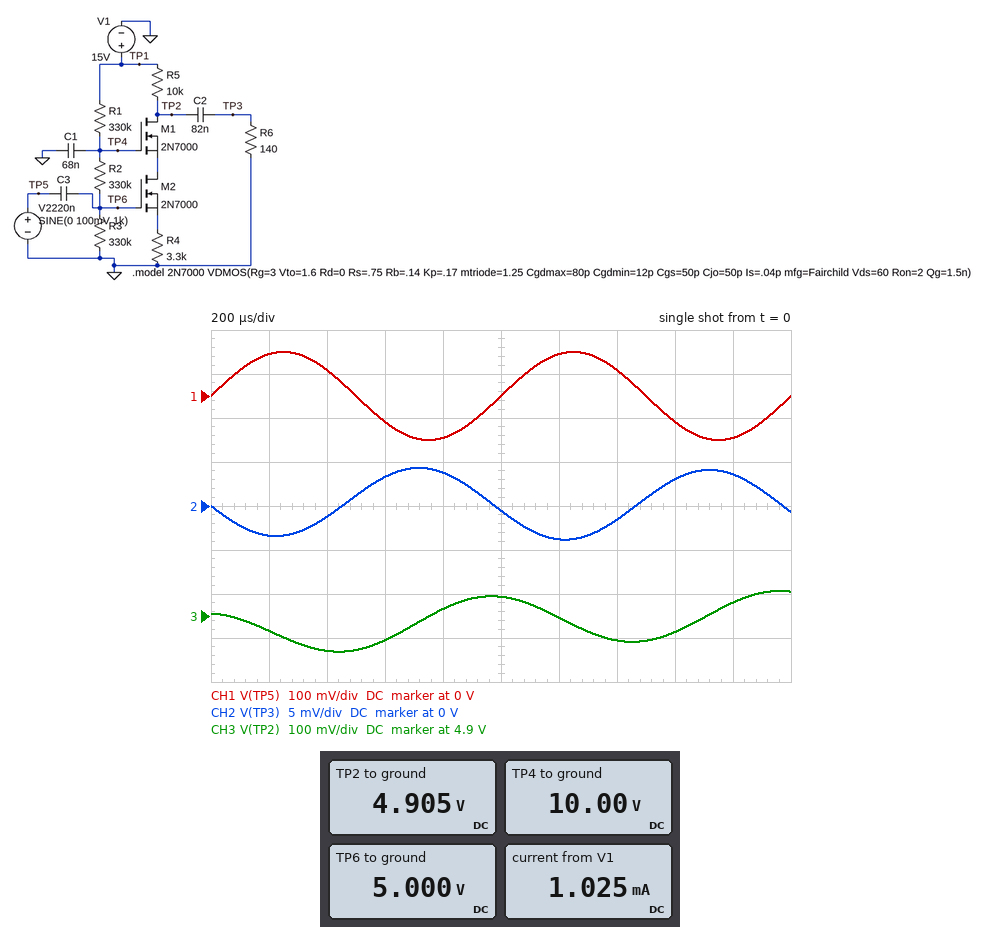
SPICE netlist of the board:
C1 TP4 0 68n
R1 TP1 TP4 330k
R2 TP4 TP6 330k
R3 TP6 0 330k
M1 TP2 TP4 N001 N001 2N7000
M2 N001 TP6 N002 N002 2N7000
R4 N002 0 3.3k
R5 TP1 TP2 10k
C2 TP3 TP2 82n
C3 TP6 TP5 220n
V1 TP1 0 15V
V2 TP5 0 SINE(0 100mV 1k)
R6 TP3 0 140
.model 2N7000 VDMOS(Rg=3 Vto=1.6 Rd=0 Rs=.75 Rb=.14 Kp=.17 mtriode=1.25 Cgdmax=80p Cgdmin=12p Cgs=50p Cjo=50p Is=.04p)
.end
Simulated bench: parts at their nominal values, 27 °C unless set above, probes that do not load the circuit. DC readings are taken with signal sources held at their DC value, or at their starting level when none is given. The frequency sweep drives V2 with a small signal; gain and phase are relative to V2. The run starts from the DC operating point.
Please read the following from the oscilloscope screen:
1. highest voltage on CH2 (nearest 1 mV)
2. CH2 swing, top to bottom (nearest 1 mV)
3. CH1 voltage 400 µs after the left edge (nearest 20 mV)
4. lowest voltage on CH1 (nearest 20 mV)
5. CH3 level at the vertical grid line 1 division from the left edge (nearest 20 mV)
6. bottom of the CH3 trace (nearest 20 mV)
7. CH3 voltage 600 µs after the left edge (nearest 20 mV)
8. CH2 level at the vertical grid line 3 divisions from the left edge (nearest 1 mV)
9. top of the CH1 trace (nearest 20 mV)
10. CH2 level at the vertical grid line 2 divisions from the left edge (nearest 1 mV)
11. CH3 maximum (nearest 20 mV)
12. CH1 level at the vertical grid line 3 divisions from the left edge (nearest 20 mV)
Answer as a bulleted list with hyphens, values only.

- 4 mV
- 8 mV
- 60 mV
- -100 mV
- 4.86 V
- 4.82 V
- 4.84 V
- 3 mV
- 100 mV
- -1 mV
- 4.96 V
- -60 mV
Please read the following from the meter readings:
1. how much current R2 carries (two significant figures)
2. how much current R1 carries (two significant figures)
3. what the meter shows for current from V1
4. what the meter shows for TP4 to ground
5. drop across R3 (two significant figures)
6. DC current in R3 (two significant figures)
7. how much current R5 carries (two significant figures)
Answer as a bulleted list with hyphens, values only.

- 15 µA
- 15 µA
- 1.025 mA
- 10.00 V
- 5.0 V
- 15 µA
- 1.0 mA
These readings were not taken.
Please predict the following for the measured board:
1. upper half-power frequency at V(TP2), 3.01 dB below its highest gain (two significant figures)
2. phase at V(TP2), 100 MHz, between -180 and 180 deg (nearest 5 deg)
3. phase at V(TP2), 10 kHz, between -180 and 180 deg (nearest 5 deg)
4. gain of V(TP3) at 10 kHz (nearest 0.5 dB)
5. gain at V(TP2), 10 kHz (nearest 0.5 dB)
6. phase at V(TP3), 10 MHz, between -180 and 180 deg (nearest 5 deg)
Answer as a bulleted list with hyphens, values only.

- 200 Hz
- 5 deg
- 125 deg
- -28.0 dB
- -23.0 dB
- 40 deg
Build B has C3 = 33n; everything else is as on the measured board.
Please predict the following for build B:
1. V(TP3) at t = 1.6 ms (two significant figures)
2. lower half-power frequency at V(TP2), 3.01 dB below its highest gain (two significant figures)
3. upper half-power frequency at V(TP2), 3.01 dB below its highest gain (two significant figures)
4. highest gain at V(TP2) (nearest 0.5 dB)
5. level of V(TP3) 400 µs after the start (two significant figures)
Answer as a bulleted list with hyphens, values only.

- 3.1 mV
- 23 Hz
- 250 Hz
- 8.0 dB
- -1.1 mV
